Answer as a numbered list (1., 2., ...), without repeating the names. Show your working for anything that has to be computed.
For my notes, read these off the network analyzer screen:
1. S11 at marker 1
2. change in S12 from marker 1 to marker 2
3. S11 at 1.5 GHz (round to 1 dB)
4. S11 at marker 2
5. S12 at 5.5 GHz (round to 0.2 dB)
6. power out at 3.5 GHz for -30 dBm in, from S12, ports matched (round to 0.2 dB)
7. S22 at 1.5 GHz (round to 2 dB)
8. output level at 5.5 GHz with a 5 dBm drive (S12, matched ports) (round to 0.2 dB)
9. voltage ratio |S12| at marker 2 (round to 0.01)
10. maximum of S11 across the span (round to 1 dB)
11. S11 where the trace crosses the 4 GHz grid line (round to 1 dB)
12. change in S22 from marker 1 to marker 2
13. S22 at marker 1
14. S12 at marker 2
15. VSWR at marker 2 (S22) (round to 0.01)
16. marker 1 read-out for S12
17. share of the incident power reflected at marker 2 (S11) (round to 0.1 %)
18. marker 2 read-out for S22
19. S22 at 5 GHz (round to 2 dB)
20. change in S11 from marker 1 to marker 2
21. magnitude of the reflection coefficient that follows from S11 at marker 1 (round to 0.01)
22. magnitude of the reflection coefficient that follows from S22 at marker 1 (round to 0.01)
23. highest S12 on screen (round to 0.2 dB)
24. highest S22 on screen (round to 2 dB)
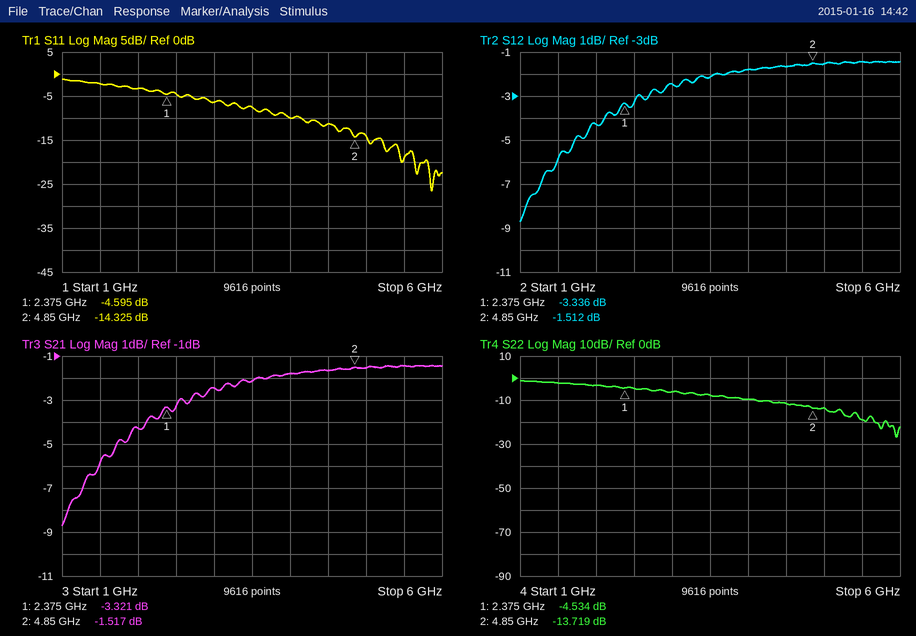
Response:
1. -4.595 dB
2. -1.512 − (-3.336) = 1.824 dB
3. -2 dB
4. -14.325 dB
5. -1.4 dB
6. -30 dBm + (-2.2 dB) = -32.2 dBm
7. -2 dB
8. 5 dBm + (-1.4 dB) = 3.6 dBm
9. 10^(-1.512/20) ≈ 0.84
10. -1 dB
11. -10 dB
12. -13.719 − (-4.534) = -9.185 dB
13. -4.534 dB
14. -1.512 dB
15. (1 + 0.2061)/(1 − 0.2061) ≈ 1.52
16. -3.336 dB
17. 10^(-14.325/10) ≈ 3.7 %
18. -13.719 dB
19. -14 dB
20. -14.325 − (-4.595) = -9.730 dB
21. 10^(-4.595/20) ≈ 0.59
22. 10^(-4.534/20) ≈ 0.59
23. -1.4 dB
24. -2 dB
